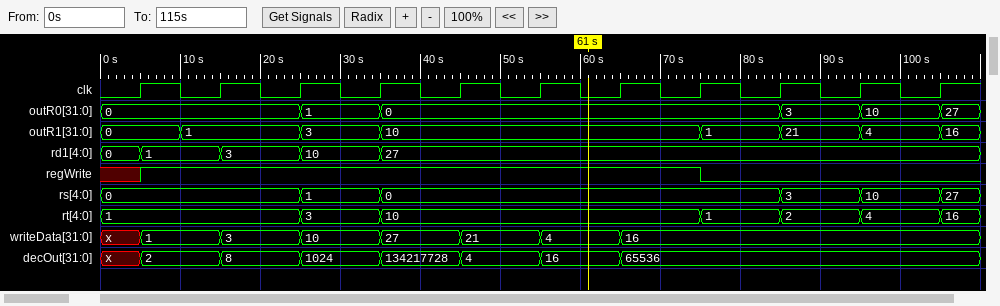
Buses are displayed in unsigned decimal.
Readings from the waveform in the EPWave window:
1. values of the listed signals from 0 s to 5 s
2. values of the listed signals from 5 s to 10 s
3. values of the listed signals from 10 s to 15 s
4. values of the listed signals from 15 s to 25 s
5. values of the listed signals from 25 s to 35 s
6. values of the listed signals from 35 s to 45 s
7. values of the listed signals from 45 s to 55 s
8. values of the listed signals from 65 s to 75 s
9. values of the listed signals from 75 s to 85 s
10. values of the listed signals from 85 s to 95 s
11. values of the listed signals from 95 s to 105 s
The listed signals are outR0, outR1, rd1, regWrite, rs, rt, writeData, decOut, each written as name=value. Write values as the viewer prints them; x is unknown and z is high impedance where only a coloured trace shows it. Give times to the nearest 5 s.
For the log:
outR0=0, outR1=0, rd1=0, regWrite=x, rs=0, rt=1, writeData=x, decOut=x
outR0=0, outR1=0, rd1=1, regWrite=1, rs=0, rt=1, writeData=1, decOut=2
outR0=0, outR1=1, rd1=1, regWrite=1, rs=0, rt=1, writeData=1, decOut=2
outR0=0, outR1=1, rd1=3, regWrite=1, rs=0, rt=1, writeData=3, decOut=8
outR0=1, outR1=3, rd1=10, regWrite=1, rs=1, rt=3, writeData=10, decOut=1024
outR0=0, outR1=10, rd1=27, regWrite=1, rs=0, rt=10, writeData=27, decOut=134217728
outR0=0, outR1=10, rd1=27, regWrite=1, rs=0, rt=10, writeData=21, decOut=4
outR0=0, outR1=10, rd1=27, regWrite=1, rs=0, rt=10, writeData=16, decOut=65536
outR0=0, outR1=1, rd1=27, regWrite=0, rs=0, rt=1, writeData=16, decOut=65536
outR0=3, outR1=21, rd1=27, regWrite=0, rs=3, rt=2, writeData=16, decOut=65536
outR0=10, outR1=4, rd1=27, regWrite=0, rs=10, rt=4, writeData=16, decOut=65536
